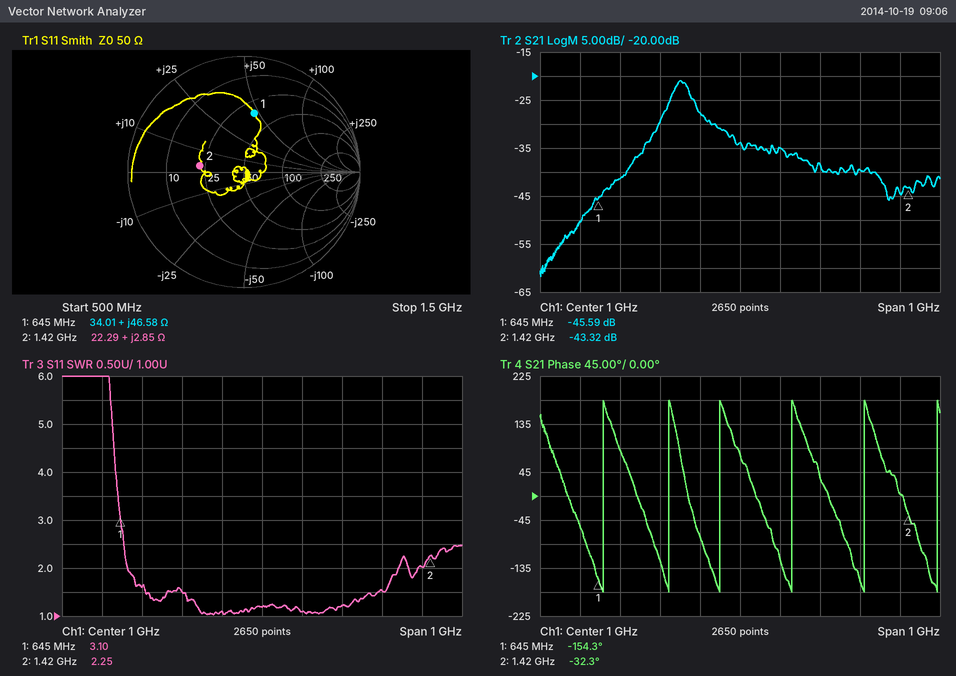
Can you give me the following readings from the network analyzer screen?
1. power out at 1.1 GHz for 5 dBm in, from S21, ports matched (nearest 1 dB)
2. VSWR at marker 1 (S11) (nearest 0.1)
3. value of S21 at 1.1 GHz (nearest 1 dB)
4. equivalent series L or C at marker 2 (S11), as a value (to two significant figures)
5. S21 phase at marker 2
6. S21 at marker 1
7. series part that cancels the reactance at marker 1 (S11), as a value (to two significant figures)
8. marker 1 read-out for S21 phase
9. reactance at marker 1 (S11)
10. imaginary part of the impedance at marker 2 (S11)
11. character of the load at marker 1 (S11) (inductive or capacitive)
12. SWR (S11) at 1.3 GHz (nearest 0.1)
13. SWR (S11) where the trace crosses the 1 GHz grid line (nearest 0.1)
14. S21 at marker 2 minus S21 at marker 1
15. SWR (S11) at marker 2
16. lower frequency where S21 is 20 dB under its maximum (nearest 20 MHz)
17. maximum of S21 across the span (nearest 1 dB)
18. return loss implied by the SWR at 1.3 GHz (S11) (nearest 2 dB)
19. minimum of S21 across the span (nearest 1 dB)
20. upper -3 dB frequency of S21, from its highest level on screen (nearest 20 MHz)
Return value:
-30 dBm
3.1
-35 dB
320 pH
-32.3°
-45.59 dB
5.3 pF
-154.3°
+46.58 Ω
+2.85 Ω
inductive
1.5
1.2
2.27 dB
2.25
700 MHz
-21 dB
14 dB
-62 dB
880 MHz
